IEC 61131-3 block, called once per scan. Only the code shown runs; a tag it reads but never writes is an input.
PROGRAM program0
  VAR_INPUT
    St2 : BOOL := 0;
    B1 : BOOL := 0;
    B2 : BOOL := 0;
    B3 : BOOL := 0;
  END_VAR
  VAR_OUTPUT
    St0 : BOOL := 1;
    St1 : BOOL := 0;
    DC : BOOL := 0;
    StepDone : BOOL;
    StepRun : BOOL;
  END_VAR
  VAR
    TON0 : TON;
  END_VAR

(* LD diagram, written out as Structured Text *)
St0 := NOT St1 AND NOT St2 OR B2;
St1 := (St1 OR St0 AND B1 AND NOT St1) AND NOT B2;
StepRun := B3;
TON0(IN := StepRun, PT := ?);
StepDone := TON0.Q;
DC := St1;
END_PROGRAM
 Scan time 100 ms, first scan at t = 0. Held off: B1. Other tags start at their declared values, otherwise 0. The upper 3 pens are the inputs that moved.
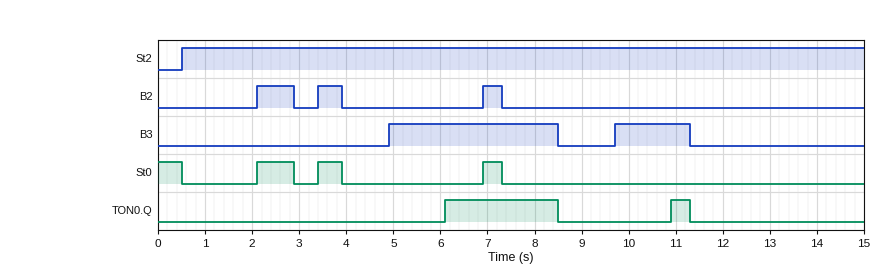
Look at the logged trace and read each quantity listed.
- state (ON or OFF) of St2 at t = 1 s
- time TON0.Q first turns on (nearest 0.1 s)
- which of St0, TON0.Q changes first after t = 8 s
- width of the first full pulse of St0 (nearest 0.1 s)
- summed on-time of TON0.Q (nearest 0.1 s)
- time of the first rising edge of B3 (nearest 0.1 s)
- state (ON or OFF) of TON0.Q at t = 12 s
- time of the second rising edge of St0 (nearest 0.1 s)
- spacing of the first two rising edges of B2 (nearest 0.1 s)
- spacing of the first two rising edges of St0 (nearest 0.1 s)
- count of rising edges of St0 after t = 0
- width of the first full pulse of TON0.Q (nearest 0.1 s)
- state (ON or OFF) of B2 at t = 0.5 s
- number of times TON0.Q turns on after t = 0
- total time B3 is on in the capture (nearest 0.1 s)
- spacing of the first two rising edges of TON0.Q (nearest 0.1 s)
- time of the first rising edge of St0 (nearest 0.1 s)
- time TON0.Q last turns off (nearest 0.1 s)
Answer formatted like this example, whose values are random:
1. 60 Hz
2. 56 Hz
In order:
1. ON
2. 6.1 s
3. TON0.Q
4. 0.8 s
5. 2.8 s
6. 4.9 s
7. OFF
8. 3.4 s
9. 1.3 s
10. 1.3 s
11. 3
12. 2.4 s
13. OFF
14. 2
15. 5.2 s
16. 4.8 s
17. 2.1 s
18. 11.3 s
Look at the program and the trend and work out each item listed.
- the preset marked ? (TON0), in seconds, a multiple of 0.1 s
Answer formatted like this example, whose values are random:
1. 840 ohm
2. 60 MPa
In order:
1. 1.2 s
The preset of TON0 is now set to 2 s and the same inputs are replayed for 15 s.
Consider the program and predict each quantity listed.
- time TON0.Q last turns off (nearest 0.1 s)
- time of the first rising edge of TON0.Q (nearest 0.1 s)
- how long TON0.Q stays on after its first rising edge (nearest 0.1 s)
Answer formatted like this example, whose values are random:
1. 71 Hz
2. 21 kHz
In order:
1. 8.5 s
2. 6.9 s
3. 1.6 s
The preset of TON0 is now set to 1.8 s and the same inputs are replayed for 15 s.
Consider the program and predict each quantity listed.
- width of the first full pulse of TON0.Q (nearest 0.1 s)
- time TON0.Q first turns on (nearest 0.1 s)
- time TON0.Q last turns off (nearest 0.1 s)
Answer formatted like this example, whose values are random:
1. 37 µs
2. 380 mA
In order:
1. 1.8 s
2. 6.7 s
3. 8.5 s
